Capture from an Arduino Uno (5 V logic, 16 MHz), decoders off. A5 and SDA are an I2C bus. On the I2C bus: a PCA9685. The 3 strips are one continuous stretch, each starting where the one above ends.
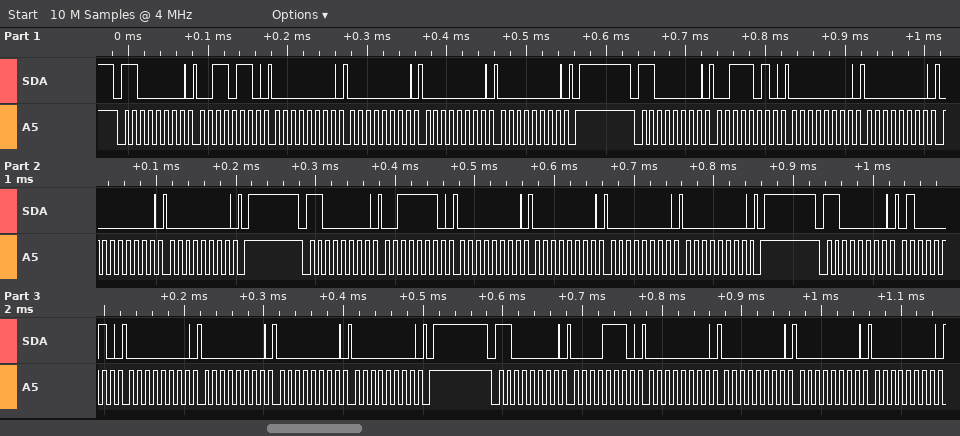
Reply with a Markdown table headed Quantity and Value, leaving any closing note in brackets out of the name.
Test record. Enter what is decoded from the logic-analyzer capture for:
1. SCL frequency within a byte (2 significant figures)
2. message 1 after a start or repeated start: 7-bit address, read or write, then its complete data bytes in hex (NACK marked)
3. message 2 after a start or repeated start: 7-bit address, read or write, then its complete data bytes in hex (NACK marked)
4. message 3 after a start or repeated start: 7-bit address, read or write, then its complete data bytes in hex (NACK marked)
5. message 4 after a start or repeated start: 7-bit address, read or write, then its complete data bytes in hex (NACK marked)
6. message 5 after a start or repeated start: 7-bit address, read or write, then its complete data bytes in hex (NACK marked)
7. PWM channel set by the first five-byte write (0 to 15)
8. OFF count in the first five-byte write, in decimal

| Quantity | Value |
|---|---|
| SCL frequency within a byte | 100 kHz |
| message 1 after a start or repeated start: 7-bit address, read or write, then its complete data bytes in hex | 0x60 write: 36 00 00 00 00 |
| message 2 after a start or repeated start: 7-bit address, read or write, then its complete data bytes in hex | 0x60 write: 3A 00 00 00 00 |
| message 3 after a start or repeated start: 7-bit address, read or write, then its complete data bytes in hex | 0x60 write: 3E 00 00 00 00 |
| message 4 after a start or repeated start: 7-bit address, read or write, then its complete data bytes in hex | 0x60 write: 42 00 00 00 00 |
| message 5 after a start or repeated start: 7-bit address, read or write, then its complete data bytes in hex | 0x60 write: 0E 00 00 00 00 |
| PWM channel set by the first five-byte write | 12 |
| OFF count in the first five-byte write, in decimal | 0 |
